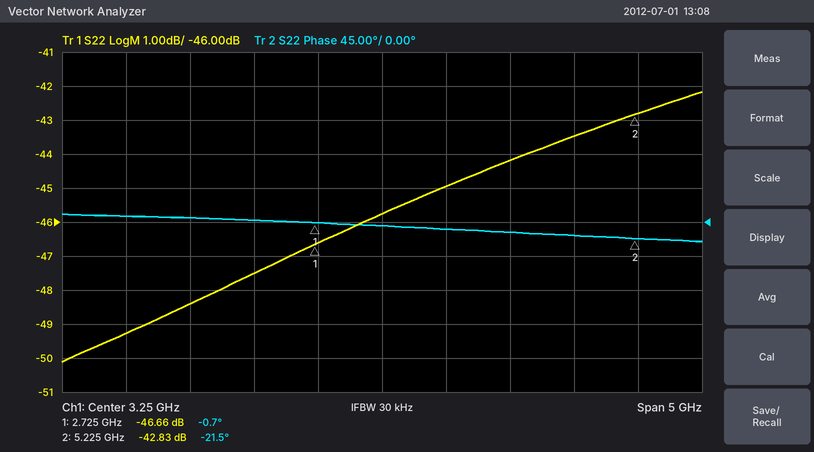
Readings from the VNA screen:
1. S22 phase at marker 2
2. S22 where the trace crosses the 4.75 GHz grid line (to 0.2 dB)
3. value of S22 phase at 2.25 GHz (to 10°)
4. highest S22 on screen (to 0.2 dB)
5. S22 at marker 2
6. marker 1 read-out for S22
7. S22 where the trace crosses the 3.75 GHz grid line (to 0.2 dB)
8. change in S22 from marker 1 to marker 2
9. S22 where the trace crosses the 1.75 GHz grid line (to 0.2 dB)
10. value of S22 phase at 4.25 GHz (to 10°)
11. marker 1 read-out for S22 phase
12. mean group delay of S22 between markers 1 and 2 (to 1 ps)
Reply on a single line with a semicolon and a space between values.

-21.5°; -43.4 dB; 0°; -42.2 dB; -42.83 dB; -46.66 dB; -45.0 dB; 3.83 dB; -48.4 dB; -10°; -0.7°; 23 ps
